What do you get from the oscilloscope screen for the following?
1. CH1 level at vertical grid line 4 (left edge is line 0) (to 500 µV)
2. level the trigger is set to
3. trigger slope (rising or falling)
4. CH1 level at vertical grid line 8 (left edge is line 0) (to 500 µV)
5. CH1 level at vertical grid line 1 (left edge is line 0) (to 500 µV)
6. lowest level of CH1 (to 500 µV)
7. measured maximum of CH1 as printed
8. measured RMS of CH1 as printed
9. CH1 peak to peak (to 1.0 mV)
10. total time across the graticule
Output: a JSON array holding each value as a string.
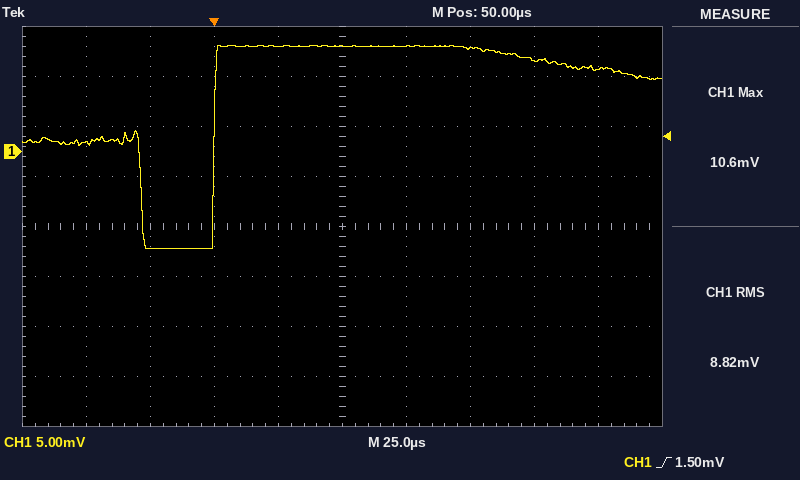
["10.5 mV", "1.50 mV", "rising", "9.0 mV", "1.0 mV", "-9.5 mV", "10.6 mV", "8.82 mV", "20.0 mV", "250 µs"]
